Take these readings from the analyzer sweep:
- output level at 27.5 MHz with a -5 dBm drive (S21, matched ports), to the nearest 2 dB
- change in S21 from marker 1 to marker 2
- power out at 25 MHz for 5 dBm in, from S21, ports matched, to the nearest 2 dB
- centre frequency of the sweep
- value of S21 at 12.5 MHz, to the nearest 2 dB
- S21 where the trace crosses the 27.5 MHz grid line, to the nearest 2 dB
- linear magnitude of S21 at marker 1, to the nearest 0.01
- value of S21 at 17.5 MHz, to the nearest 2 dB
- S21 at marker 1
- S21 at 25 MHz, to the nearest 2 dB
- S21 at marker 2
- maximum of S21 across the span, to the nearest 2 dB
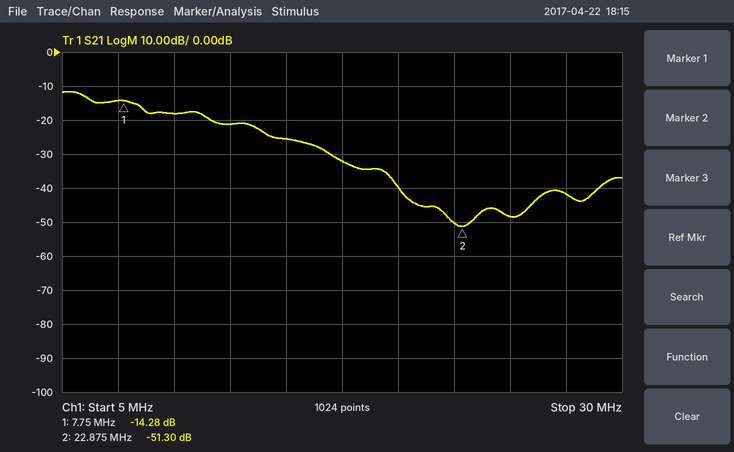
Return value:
-46 dBm
-37.02 dB
-44 dBm
17.5 MHz
-22 dB
-42 dB
0.19
-32 dB
-14.28 dB
-48 dB
-51.30 dB
-12 dB
